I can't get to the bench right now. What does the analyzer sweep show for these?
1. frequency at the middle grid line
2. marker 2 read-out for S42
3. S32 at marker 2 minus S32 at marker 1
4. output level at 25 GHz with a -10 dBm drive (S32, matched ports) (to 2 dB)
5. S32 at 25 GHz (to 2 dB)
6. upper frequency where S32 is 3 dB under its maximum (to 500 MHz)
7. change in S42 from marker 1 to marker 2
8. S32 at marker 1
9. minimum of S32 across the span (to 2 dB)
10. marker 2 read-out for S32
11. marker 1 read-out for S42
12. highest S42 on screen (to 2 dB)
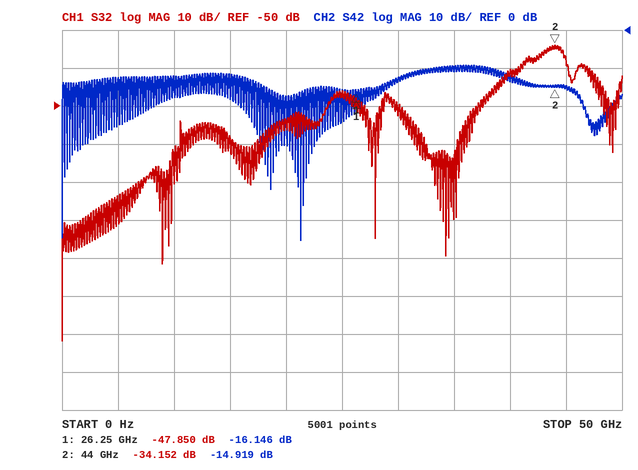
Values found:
25 GHz
-14.919 dB
13.698 dB
-56 dBm
-46 dB
45.0 GHz
1.227 dB
-47.850 dB
-112 dB
-34.152 dB
-16.146 dB
-10 dB
